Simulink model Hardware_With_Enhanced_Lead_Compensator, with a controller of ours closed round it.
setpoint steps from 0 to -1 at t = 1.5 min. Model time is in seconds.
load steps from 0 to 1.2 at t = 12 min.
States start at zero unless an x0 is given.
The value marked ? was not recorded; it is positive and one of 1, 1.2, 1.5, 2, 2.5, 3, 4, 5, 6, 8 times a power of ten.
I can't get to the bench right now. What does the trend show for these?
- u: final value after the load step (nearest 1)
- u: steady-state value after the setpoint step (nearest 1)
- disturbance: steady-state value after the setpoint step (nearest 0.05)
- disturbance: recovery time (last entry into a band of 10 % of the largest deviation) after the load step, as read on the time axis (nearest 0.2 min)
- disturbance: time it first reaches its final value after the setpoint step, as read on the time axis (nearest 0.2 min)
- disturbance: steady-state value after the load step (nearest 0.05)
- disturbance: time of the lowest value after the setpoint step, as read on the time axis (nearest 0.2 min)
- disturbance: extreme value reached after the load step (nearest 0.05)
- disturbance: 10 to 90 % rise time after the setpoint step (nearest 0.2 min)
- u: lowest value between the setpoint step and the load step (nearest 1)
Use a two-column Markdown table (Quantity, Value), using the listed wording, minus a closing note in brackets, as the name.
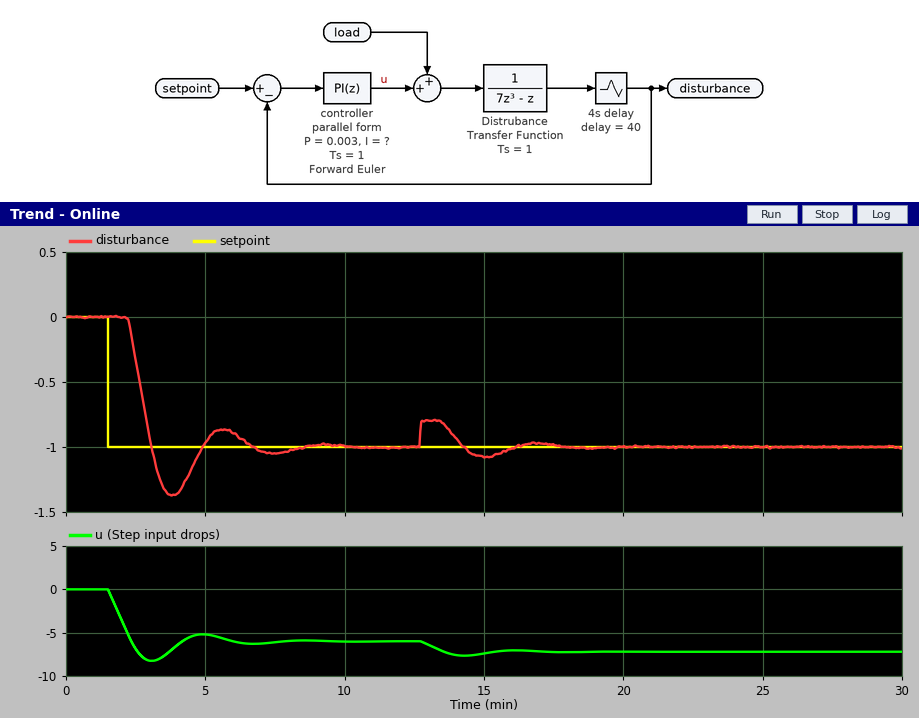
| Quantity | Value |
|---|---|
| u: final value after the load step | -7 |
| u: steady-state value after the setpoint step | -6 |
| disturbance: steady-state value after the setpoint step | -1.00 |
| disturbance: recovery time (last entry into a band of 10 % of the largest deviation) after the load step, as read on the time axis | 17.2 min |
| disturbance: time it first reaches its final value after the setpoint step, as read on the time axis | 3.0 min |
| disturbance: steady-state value after the load step | -1.00 |
| disturbance: time of the lowest value after the setpoint step, as read on the time axis | 3.8 min |
| disturbance: extreme value reached after the load step | -0.80 |
| disturbance: 10 to 90 % rise time after the setpoint step | 0.6 min |
| u: lowest value between the setpoint step and the load step | -8 |
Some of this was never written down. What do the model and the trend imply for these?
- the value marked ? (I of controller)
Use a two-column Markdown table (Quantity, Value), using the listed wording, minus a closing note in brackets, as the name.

| Quantity | Value |
|---|---|
| the value marked ? | 0.12 |
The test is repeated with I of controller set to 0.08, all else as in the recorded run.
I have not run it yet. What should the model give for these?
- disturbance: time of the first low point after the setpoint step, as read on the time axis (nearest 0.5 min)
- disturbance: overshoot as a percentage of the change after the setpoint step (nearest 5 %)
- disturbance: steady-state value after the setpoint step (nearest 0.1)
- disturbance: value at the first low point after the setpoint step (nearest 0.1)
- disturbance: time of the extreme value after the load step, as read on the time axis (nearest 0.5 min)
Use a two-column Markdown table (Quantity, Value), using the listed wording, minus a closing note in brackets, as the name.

| Quantity | Value |
|---|---|
| disturbance: time of the first low point after the setpoint step, as read on the time axis | 4.5 min |
| disturbance: overshoot as a percentage of the change after the setpoint step | 10 % |
| disturbance: steady-state value after the setpoint step | -1.0 |
| disturbance: value at the first low point after the setpoint step | -1.1 |
| disturbance: time of the extreme value after the load step, as read on the time axis | 13.0 min |
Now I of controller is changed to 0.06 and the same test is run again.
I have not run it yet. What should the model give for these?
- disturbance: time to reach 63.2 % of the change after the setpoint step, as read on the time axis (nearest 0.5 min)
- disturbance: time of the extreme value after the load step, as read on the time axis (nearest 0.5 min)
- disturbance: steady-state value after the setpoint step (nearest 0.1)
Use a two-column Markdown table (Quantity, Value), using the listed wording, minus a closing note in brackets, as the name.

| Quantity | Value |
|---|---|
| disturbance: time to reach 63.2 % of the change after the setpoint step, as read on the time axis | 3.5 min |
| disturbance: time of the extreme value after the load step, as read on the time axis | 13.0 min |
| disturbance: steady-state value after the setpoint step | -1.0 |
